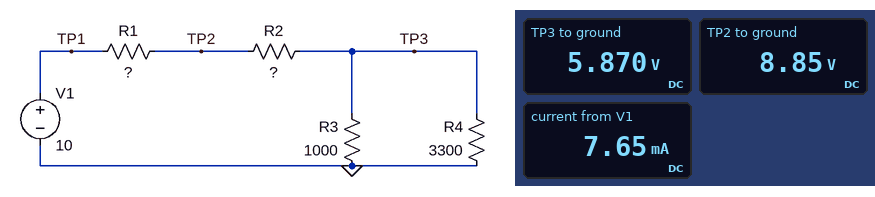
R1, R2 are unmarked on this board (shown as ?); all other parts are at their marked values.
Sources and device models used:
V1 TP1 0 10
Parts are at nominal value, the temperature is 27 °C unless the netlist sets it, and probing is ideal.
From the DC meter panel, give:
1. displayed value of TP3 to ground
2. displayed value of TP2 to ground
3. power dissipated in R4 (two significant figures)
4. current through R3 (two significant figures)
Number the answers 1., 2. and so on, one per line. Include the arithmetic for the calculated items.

1. 5.870 V
2. 8.85 V
3. (5.87 V)^2 / 3.3 kΩ = 10 mW
4. (5.87 V) / 1 kΩ = 5.9 mA
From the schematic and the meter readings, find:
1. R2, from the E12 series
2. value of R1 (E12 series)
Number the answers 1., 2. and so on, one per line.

1. 390 Ω
2. 150 Ω
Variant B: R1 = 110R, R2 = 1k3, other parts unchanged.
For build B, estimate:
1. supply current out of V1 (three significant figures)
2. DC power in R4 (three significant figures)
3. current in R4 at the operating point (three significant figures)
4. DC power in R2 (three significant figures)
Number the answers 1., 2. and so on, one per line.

1. 4.59 mA
2. 3.76 mW
3. 1.07 mA
4. 27.4 mW
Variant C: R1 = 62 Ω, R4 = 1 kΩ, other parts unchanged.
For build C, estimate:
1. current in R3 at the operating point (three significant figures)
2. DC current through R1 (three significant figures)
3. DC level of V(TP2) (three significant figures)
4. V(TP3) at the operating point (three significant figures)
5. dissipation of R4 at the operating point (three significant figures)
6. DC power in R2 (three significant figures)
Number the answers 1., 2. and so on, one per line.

1. 5.25 mA
2. 10.5 mA
3. 9.35 V
4. 5.25 V
5. 27.6 mW
6. 43.0 mW
